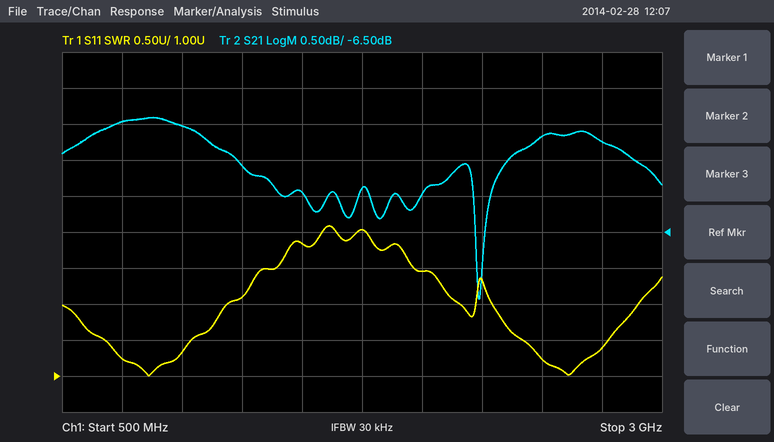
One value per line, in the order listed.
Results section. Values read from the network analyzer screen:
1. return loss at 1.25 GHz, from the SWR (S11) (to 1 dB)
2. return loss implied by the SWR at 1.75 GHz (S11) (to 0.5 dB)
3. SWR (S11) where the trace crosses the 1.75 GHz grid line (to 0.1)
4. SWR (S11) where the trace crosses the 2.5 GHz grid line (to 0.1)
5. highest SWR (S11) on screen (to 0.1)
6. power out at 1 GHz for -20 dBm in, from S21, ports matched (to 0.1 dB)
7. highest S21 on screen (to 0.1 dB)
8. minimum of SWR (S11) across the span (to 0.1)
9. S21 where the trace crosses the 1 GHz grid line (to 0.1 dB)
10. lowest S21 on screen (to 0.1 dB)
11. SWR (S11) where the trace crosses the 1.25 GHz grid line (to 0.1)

9 dB
6.0 dB
3.0
1.2
3.1
-25.0 dBm
-4.9 dB
1.0
-5.0 dB
-7.4 dB
2.1
